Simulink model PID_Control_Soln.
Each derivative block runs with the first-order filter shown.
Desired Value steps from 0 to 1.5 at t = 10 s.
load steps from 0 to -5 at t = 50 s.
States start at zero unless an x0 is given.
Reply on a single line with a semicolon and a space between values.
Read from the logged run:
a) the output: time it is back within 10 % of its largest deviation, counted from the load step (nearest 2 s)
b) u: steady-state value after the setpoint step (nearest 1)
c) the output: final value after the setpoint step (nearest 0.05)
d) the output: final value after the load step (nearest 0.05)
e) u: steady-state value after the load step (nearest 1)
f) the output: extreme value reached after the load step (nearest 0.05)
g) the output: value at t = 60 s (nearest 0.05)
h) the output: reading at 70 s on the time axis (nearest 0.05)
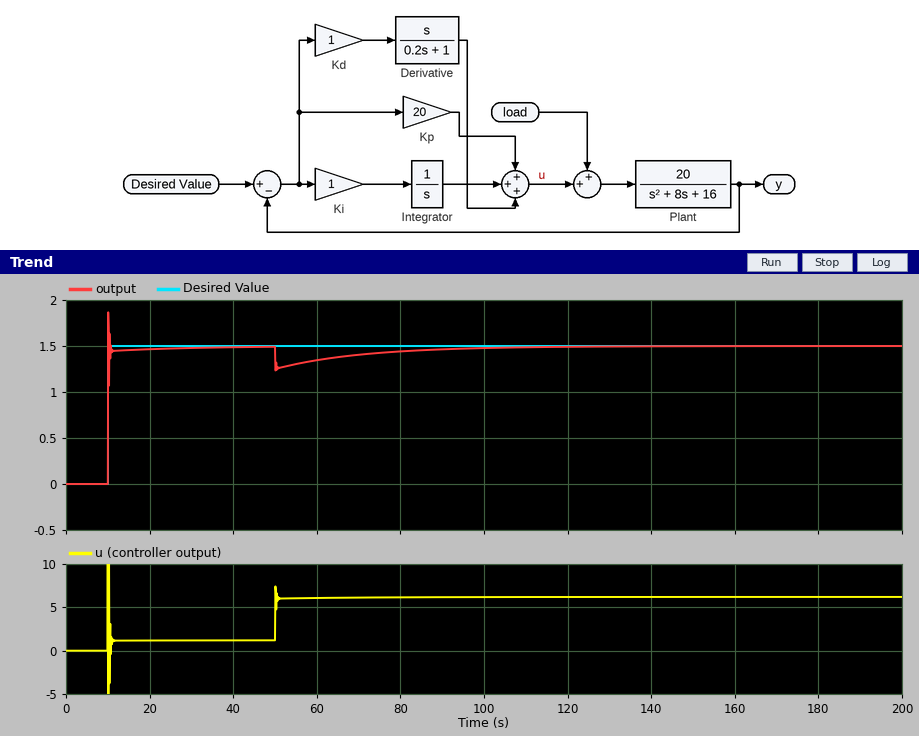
48 s; 1; 1.50; 1.50; 6; 1.25; 1.35; 1.40
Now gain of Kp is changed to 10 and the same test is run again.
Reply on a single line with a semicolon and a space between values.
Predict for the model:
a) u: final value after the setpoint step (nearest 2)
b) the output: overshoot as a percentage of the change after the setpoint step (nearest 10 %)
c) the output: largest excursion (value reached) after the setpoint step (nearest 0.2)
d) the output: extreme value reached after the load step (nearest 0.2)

2; 30 %; 2.0; 1.0
